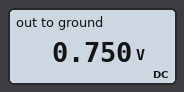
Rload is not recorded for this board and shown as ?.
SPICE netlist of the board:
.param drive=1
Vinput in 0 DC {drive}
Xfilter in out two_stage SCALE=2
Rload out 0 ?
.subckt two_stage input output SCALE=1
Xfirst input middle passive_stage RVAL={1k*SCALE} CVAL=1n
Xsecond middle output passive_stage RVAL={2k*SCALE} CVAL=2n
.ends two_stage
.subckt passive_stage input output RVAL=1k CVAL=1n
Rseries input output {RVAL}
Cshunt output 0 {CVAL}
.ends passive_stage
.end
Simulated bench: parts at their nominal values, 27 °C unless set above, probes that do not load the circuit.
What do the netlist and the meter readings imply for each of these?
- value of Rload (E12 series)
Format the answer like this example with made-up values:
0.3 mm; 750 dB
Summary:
18 kΩ
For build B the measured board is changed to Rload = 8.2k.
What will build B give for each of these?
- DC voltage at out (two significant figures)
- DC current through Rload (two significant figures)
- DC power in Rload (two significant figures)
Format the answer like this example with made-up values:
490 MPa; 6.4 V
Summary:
580 mV; 70 µA; 41 µW
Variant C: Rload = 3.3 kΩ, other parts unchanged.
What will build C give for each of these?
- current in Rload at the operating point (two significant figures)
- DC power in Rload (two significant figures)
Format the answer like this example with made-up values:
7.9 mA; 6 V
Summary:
110 µA; 38 µW
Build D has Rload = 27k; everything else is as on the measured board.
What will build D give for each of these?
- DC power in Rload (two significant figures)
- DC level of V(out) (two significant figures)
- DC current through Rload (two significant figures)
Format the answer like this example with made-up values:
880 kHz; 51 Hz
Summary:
25 µW; 820 mV; 30 µA
